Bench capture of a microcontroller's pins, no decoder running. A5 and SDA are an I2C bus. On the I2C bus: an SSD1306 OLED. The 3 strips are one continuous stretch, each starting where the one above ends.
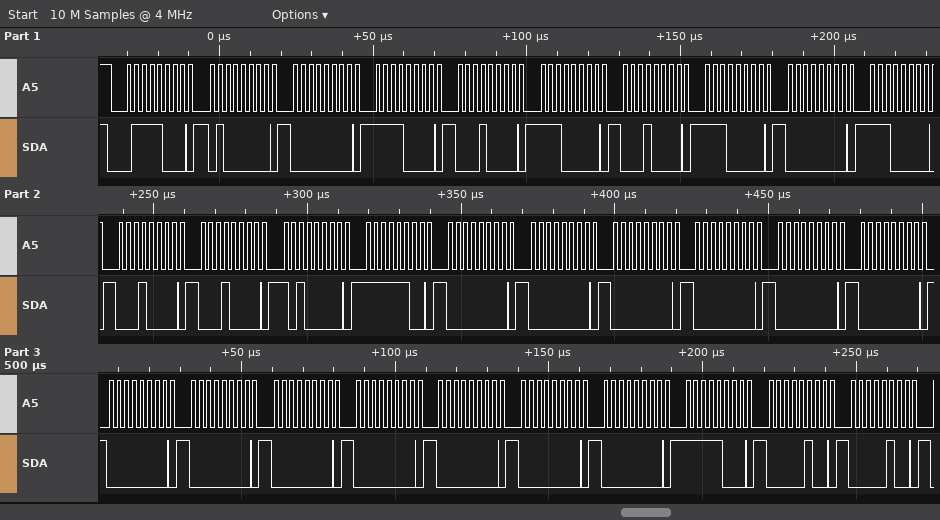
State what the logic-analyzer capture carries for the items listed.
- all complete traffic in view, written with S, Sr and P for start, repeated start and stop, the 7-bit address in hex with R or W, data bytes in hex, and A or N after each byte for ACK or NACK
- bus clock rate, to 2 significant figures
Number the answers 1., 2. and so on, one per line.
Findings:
1. S 3CW A 40 A 00 A F0 A 10 A E0 A 10 A E0 A 00 A E0 A 10 A 10 A A0 A FC A 00 A 00 A 00 A 00 A 00 A 00 A 00 A 00 A 00 A 00 A 00 A 00 A 00 A F8 A 04 A 04 A
2. 400 kHz
